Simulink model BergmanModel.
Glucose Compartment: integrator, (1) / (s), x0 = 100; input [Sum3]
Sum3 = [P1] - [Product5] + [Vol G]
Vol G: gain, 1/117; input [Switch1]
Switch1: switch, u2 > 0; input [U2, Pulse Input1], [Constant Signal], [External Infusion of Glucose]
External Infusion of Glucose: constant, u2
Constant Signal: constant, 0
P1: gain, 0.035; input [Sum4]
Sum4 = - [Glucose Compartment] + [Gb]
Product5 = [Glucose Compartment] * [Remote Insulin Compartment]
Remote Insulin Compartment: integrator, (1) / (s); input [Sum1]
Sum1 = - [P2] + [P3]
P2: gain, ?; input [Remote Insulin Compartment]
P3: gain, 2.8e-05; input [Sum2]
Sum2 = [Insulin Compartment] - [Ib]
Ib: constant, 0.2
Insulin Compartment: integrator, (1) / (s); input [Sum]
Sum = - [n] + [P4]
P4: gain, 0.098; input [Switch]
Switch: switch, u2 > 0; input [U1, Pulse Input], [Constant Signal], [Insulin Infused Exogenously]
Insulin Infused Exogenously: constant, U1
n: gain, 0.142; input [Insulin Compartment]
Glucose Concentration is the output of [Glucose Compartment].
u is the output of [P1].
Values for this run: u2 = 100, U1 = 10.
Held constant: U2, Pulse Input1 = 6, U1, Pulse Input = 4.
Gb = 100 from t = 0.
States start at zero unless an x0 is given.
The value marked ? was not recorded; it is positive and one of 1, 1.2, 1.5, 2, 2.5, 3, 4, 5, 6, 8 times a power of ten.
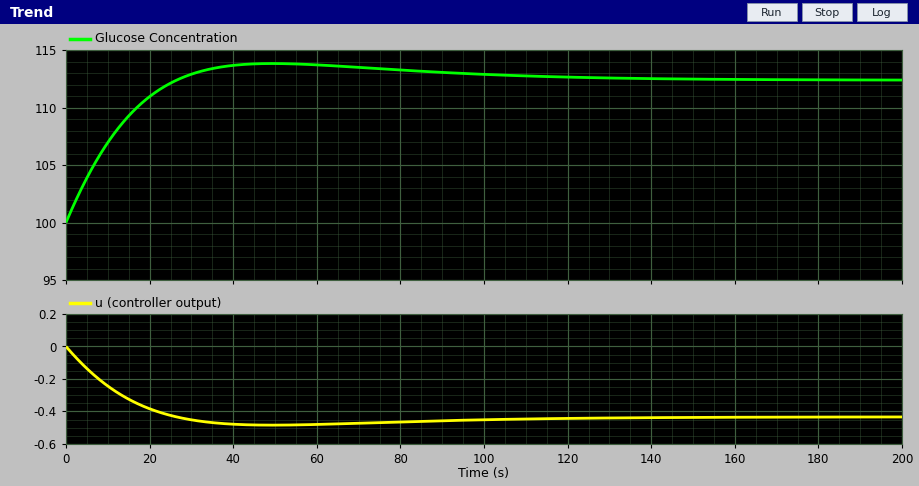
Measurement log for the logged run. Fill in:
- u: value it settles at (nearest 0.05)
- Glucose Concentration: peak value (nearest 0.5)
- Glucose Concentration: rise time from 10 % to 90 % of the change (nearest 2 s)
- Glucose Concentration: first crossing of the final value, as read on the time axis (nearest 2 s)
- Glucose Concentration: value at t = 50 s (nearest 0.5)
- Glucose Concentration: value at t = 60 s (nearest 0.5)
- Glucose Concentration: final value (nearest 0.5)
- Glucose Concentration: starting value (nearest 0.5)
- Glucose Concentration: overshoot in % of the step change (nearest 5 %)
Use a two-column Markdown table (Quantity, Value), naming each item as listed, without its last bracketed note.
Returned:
| Quantity | Value |
|---|---|
| u: value it settles at | -0.45 |
| Glucose Concentration: peak value | 114.0 |
| Glucose Concentration: rise time from 10 % to 90 % of the change | 20 s |
| Glucose Concentration: first crossing of the final value, as read on the time axis | 26 s |
| Glucose Concentration: value at t = 50 s | 114.0 |
| Glucose Concentration: value at t = 60 s | 113.5 |
| Glucose Concentration: final value | 112.5 |
| Glucose Concentration: starting value | 100.0 |
| Glucose Concentration: overshoot in % of the step change | 10 % |
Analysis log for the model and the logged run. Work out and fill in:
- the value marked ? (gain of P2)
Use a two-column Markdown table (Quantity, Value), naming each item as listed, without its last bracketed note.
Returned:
| Quantity | Value |
|---|---|
| the value marked ? | 0.05 |
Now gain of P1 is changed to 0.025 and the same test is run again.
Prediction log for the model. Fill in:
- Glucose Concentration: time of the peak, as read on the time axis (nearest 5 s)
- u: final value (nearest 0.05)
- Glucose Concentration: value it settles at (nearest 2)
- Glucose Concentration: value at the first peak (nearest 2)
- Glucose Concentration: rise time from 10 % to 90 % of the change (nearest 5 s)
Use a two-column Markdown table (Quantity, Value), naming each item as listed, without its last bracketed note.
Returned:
| Quantity | Value |
|---|---|
| Glucose Concentration: time of the peak, as read on the time axis | 70 s |
| u: final value | -0.40 |
| Glucose Concentration: value it settles at | 116 |
| Glucose Concentration: value at the first peak | 118 |
| Glucose Concentration: rise time from 10 % to 90 % of the change | 30 s |
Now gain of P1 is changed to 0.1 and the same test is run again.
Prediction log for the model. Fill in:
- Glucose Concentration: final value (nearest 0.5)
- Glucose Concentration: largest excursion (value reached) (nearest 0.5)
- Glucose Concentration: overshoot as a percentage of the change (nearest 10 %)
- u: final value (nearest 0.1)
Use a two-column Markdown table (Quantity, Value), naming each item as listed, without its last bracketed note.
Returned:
| Quantity | Value |
|---|---|
| Glucose Concentration: final value | 104.5 |
| Glucose Concentration: largest excursion (value reached) | 106.5 |
| Glucose Concentration: overshoot as a percentage of the change | 40 % |
| u: final value | -0.5 |
